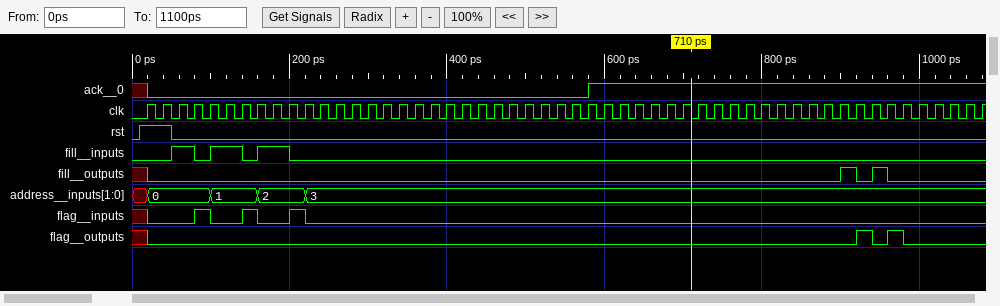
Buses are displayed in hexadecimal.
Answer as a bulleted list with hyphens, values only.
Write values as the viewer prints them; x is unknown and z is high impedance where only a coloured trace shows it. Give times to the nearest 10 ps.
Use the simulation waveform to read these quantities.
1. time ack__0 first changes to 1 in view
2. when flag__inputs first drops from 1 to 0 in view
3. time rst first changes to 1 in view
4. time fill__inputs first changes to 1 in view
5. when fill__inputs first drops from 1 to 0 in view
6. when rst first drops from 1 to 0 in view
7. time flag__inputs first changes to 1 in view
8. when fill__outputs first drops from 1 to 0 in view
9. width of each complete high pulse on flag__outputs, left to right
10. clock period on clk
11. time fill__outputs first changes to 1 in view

- 580 ps
- 100 ps
- 10 ps
- 50 ps
- 80 ps
- 50 ps
- 80 ps
- 920 ps
- 20 ps, 20 ps
- 20 ps
- 900 ps
